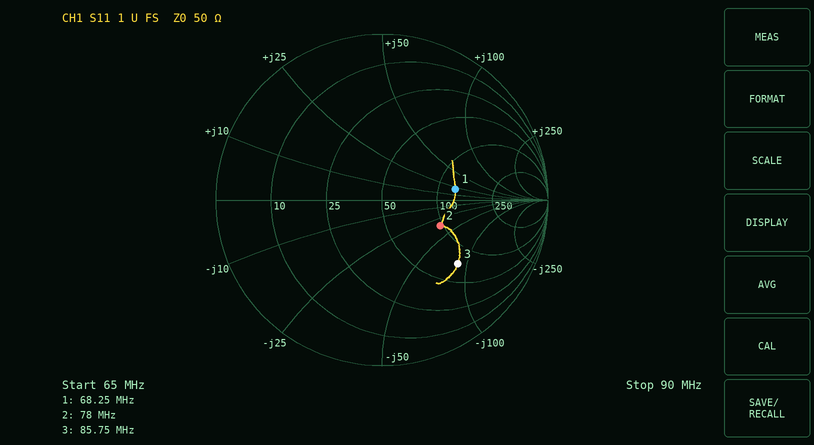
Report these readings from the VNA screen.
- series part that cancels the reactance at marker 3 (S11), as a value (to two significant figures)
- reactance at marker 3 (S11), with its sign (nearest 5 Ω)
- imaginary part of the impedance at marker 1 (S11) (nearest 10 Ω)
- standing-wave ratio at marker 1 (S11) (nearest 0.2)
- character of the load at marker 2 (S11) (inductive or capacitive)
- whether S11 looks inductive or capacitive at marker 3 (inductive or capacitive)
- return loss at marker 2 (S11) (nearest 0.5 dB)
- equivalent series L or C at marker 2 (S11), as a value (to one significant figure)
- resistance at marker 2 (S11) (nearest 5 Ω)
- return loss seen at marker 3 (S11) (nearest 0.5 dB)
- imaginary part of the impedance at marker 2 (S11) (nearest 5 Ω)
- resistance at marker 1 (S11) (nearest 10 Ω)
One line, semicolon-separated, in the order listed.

160 nH; -85 Ω; +20 Ω; 2.6; capacitive; capacitive; 8.5 dB; 60 pF; 95 Ω; 4.5 dB; -35 Ω; 130 Ω
